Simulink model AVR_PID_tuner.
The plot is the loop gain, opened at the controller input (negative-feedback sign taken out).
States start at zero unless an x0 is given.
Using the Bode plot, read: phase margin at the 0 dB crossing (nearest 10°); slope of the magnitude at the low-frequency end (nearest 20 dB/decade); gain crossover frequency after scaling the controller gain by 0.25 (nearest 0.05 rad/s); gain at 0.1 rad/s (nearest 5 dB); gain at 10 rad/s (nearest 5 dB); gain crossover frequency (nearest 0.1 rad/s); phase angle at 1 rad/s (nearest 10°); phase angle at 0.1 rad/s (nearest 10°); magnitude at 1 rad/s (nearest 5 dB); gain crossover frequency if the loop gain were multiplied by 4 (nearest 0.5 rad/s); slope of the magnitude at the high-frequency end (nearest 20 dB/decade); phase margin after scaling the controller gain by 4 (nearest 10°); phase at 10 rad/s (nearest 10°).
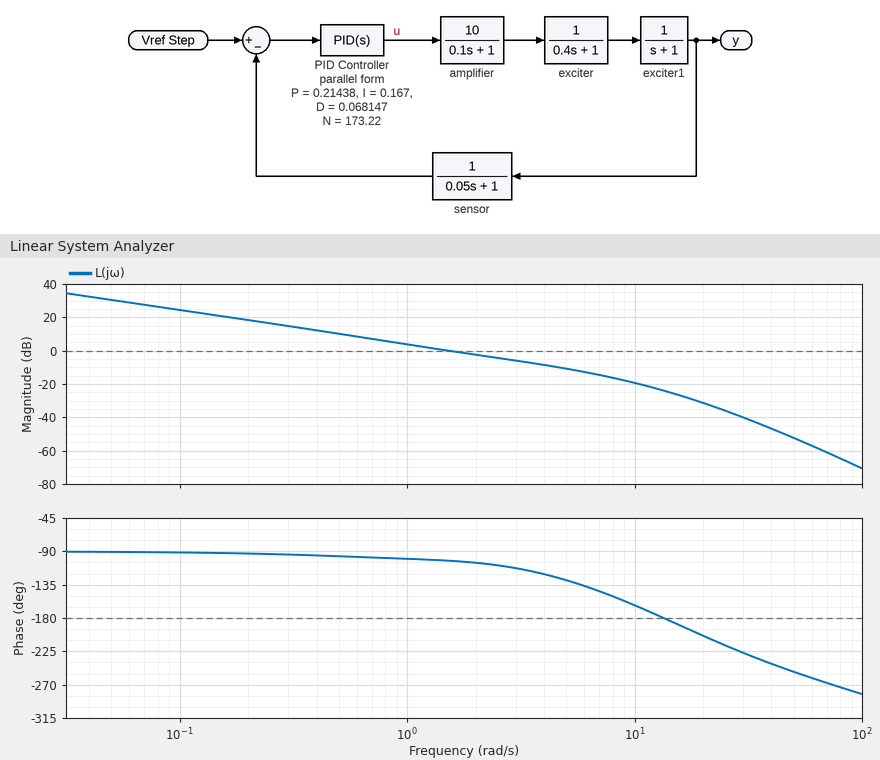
80°
-20 dB/decade
0.40 rad/s
25 dB
-20 dB
1.5 rad/s
-100°
-90°
5 dB
5.5 rad/s
-60 dB/decade
50°
-160°
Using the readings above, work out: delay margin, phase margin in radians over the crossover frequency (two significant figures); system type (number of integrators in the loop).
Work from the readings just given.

0.93 s
1
